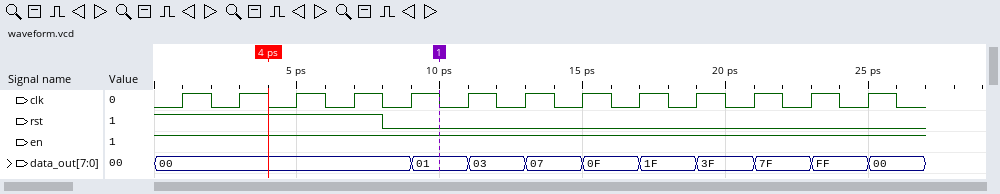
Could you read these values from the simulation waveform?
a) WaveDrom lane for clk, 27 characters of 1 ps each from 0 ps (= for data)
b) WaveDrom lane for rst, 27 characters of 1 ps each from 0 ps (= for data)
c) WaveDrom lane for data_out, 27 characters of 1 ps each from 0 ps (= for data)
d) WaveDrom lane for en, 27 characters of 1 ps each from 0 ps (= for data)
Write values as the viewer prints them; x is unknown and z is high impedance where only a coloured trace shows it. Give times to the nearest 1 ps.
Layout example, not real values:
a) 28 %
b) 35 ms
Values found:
a) {name: 'clk', wave: '010101010101010101010101010'}
b) {name: 'rst', wave: '1.......0..................'}
c) {name: 'data_out', wave: '=........=.=.=.=.=.=.=.=.=.', data: '00 01 03 07 0F 1F 3F 7F FF 00'}
d) {name: 'en', wave: '1..........................'}
